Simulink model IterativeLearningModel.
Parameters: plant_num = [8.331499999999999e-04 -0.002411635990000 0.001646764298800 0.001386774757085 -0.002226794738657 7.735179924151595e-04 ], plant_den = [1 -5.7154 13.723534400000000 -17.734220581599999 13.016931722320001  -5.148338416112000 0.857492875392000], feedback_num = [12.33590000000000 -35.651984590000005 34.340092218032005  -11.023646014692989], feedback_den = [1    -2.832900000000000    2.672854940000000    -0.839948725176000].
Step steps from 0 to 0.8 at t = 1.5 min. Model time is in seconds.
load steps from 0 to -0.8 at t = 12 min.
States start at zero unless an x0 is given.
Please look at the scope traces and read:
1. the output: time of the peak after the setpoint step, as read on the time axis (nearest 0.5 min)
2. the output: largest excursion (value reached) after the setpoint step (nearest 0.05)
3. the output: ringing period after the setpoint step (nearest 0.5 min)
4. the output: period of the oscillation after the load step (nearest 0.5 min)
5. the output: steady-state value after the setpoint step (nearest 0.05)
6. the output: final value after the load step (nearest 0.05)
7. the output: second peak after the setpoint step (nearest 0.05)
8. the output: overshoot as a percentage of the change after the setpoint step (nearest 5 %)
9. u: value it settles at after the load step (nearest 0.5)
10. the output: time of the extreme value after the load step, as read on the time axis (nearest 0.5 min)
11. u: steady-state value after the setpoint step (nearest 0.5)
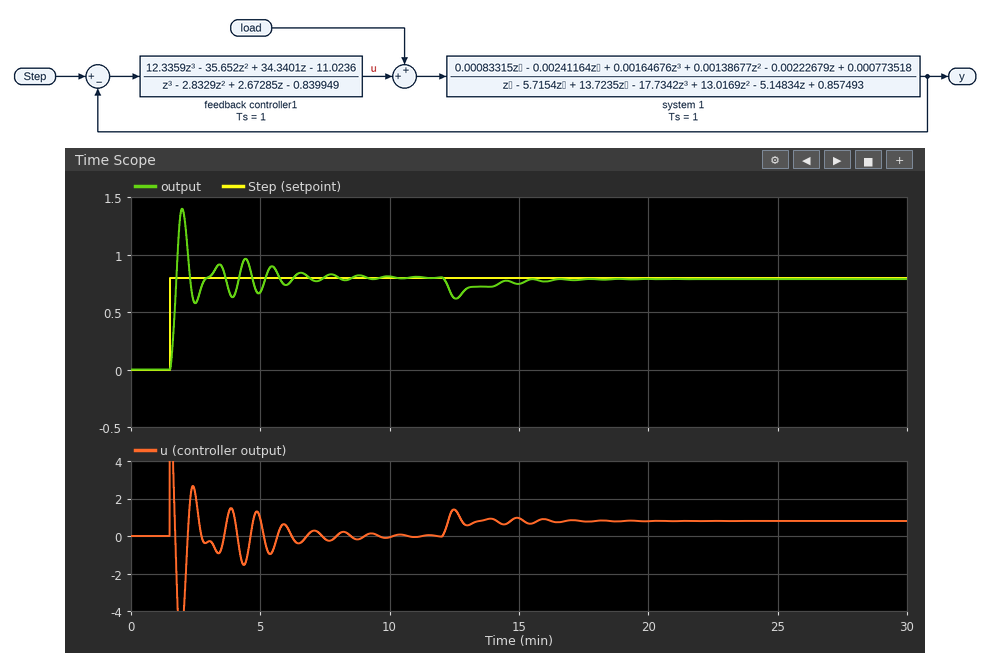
2.0 min
1.40
1.5 min
2.5 min
0.80
0.80
0.90
75 %
1.0
12.5 min
0.0
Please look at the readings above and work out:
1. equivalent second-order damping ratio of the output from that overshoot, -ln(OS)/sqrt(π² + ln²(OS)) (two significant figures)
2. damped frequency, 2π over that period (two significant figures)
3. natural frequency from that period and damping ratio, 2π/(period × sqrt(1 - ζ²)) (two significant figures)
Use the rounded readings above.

0.091
4.2 rad/min
4.2 rad/min
